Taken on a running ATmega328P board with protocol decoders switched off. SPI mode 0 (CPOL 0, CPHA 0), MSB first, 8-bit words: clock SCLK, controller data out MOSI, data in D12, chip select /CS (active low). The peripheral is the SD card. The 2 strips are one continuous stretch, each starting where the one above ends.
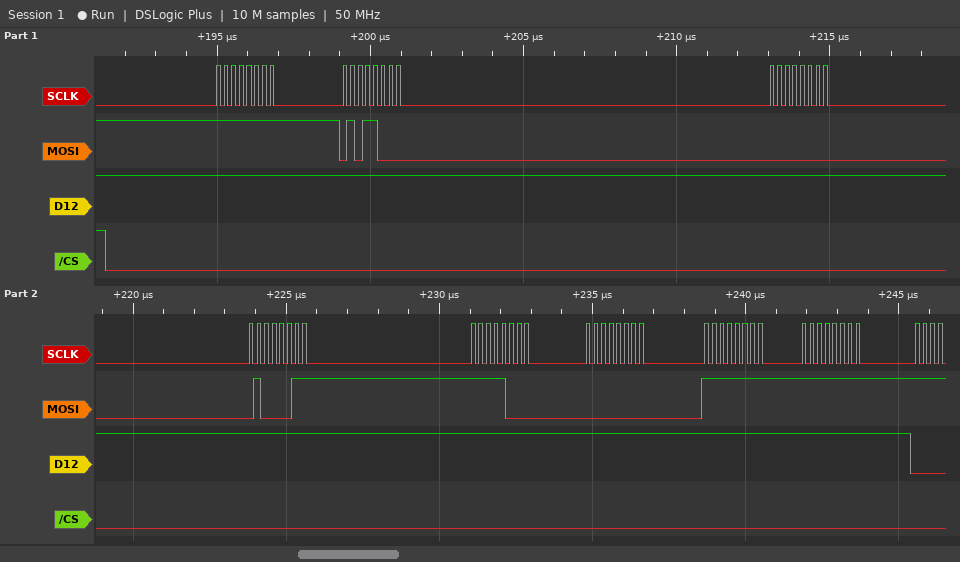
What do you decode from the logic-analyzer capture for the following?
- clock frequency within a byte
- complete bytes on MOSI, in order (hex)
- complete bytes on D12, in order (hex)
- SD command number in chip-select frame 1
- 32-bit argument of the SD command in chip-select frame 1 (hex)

4 MHz
FF 58 00 43 F8 00 FF FF
FF FF FF FF FF FF FF FF
CMD24
0x0043F800
